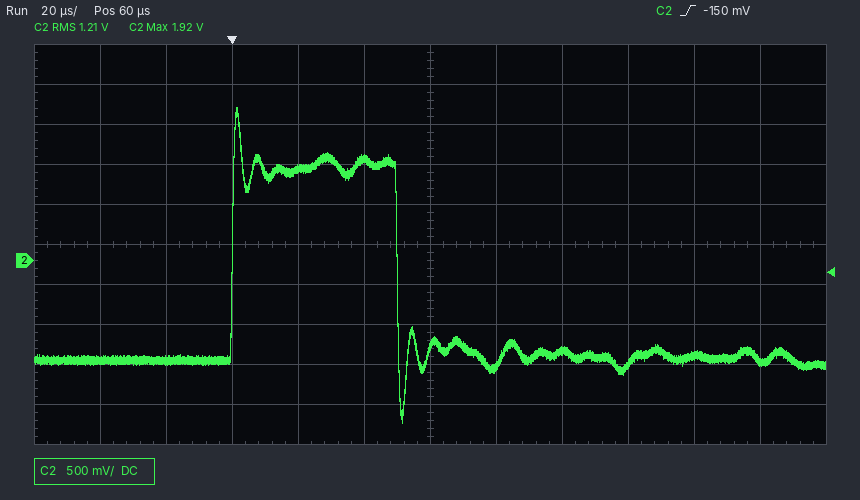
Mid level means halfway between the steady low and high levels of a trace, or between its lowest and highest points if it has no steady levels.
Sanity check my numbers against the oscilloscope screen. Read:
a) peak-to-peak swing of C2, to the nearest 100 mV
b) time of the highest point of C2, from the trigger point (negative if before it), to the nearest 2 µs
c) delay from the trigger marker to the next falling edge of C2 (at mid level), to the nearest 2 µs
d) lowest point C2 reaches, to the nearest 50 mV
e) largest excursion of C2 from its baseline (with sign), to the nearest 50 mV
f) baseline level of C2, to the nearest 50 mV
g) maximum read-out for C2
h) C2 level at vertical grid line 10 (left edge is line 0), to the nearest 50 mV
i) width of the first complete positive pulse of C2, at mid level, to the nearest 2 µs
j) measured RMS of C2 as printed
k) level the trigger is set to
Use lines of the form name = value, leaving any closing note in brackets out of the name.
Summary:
peak-to-peak swing of C2, to the nearest 100 mV = 3.90 V
time of the highest point of C2, from the trigger point (negative if before it), to the nearest 2 µs = +2 µs
delay from the trigger marker to the next falling edge of C2 (at mid level), to the nearest 2 µs = 50 µs
lowest point C2 reaches, to the nearest 50 mV = -2.00 V
largest excursion of C2 from its baseline (with sign), to the nearest 50 mV = +3.15 V
baseline level of C2, to the nearest 50 mV = -1.25 V
maximum read-out for C2 = 1.92 V
C2 level at vertical grid line 10 (left edge is line 0), to the nearest 50 mV = -1.20 V
width of the first complete positive pulse of C2, at mid level, to the nearest 2 µs = 50 µs
measured RMS of C2 as printed = 1.21 V
level the trigger is set to = -150 mV
